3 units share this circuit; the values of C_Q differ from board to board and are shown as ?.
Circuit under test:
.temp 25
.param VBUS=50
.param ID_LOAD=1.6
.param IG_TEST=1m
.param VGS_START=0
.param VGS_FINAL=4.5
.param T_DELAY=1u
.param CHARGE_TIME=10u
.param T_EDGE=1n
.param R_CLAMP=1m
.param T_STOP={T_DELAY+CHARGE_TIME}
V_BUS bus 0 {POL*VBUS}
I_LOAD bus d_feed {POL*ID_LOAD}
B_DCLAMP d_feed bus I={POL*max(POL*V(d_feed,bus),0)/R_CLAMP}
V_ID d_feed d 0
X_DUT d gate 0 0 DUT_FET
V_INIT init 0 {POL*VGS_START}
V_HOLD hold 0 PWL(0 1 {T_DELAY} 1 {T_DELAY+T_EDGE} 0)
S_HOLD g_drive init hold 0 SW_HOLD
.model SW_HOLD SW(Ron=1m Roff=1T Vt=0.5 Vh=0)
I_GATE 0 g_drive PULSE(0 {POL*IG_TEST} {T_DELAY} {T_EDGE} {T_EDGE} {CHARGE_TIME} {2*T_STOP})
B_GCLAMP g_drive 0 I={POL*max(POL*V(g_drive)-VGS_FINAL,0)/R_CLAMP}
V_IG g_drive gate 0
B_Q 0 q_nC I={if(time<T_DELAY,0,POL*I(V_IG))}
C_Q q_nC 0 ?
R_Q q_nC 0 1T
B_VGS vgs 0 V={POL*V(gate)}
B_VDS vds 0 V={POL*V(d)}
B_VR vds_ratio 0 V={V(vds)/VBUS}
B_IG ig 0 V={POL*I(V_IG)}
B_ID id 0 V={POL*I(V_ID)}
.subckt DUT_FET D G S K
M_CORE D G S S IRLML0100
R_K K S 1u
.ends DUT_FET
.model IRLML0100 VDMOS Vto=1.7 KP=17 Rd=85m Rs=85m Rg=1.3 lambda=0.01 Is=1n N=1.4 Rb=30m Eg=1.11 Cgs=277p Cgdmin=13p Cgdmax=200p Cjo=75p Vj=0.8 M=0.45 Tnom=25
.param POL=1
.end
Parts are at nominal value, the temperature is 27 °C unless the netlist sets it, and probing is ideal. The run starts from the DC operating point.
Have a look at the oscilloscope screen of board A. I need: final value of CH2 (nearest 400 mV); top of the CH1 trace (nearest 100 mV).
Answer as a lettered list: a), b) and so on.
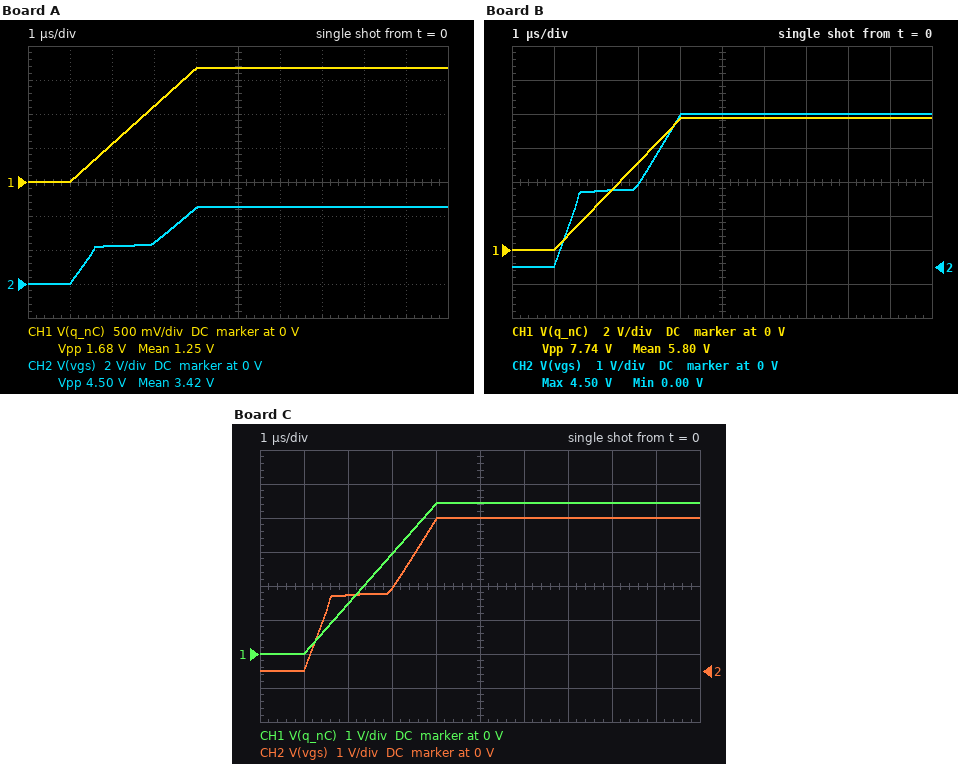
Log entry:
a) 4.4 V
b) 1.7 V
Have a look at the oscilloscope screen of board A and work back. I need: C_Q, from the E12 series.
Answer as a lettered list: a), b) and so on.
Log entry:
a) 1.8 nF
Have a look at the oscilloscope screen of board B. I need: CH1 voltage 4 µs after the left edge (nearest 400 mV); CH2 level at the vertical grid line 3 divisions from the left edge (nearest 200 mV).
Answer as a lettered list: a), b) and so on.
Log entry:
a) 7.6 V
b) 2.4 V
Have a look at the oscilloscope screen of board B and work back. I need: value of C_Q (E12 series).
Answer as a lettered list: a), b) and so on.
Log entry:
a) 390 pF
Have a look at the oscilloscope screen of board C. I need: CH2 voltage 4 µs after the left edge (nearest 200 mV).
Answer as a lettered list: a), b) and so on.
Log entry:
a) 4.4 V
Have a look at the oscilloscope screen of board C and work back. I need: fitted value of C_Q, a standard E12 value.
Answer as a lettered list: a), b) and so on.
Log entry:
a) 680 pF
